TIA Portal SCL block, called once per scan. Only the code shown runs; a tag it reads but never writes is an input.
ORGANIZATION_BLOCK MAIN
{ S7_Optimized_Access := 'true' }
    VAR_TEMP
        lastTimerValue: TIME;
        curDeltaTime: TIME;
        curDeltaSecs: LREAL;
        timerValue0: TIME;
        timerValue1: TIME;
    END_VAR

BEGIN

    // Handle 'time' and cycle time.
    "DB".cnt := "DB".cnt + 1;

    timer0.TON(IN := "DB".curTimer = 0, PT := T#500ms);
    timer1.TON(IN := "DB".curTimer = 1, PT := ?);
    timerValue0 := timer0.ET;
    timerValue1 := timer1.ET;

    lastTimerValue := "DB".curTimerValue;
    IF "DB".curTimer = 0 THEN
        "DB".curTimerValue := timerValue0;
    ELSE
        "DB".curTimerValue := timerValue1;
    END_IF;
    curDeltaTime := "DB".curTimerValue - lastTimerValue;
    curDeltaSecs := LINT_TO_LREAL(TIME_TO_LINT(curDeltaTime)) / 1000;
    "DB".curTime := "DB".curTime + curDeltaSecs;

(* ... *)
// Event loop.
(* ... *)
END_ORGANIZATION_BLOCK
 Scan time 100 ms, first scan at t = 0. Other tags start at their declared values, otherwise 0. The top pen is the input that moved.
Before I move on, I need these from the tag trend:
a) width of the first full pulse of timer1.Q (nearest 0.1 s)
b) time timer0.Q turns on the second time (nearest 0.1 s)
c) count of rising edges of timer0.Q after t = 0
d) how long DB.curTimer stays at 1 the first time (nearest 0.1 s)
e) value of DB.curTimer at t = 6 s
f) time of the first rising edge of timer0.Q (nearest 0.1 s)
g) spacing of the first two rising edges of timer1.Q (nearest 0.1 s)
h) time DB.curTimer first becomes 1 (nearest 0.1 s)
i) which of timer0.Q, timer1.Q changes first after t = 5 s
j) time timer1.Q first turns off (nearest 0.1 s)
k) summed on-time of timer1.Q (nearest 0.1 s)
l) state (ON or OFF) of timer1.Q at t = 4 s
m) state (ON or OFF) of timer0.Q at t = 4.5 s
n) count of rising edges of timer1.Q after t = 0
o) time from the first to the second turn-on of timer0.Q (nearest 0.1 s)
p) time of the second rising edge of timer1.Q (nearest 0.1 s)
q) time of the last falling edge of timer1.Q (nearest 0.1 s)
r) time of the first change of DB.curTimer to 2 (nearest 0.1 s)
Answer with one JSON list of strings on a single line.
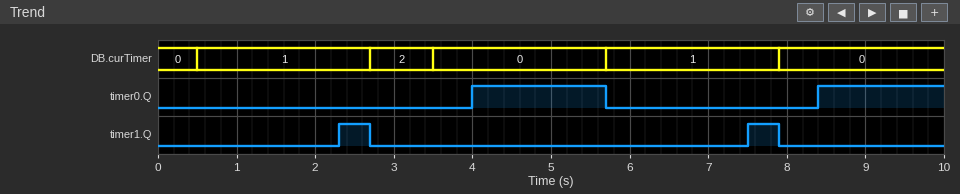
["0.4 s", "8.4 s", "2", "2.2 s", "1", "4.0 s", "5.2 s", "0.5 s", "timer0.Q", "2.7 s", "0.8 s", "OFF", "ON", "2", "4.4 s", "7.5 s", "7.9 s", "2.7 s"]
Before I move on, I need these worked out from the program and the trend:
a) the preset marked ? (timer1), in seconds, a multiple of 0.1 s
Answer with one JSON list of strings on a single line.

["1.8 s"]
